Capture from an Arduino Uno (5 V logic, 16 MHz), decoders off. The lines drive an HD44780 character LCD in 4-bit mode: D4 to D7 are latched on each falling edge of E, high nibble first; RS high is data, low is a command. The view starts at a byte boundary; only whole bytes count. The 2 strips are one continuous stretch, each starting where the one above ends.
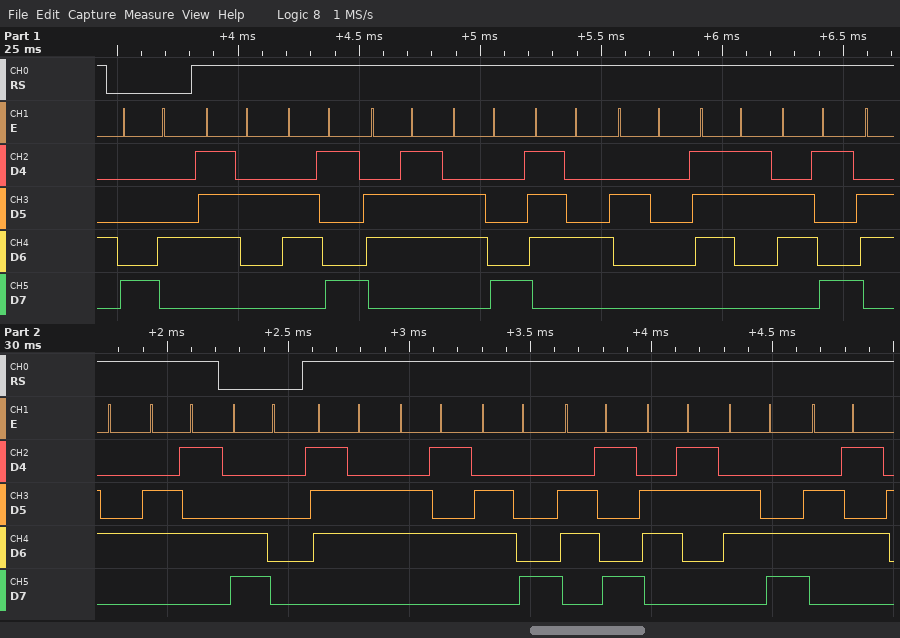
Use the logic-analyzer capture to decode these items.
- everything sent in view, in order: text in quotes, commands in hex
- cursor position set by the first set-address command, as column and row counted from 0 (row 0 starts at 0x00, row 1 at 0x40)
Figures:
0x84 "right side" 0xC0 "vehicle"
column 4, row 0
